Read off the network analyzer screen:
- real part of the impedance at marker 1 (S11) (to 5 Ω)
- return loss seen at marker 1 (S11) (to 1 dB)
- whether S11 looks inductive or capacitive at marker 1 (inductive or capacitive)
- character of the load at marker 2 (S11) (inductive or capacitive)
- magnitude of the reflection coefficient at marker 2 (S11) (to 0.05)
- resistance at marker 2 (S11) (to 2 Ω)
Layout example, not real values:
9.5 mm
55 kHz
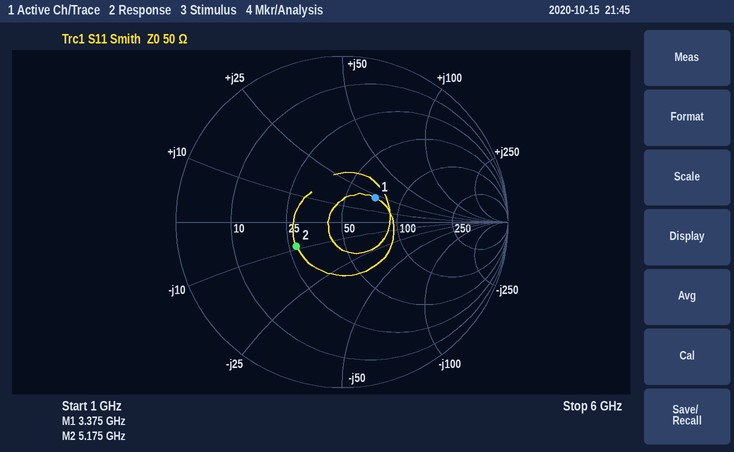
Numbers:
70 Ω
12 dB
inductive
capacitive
0.30
28 Ω
